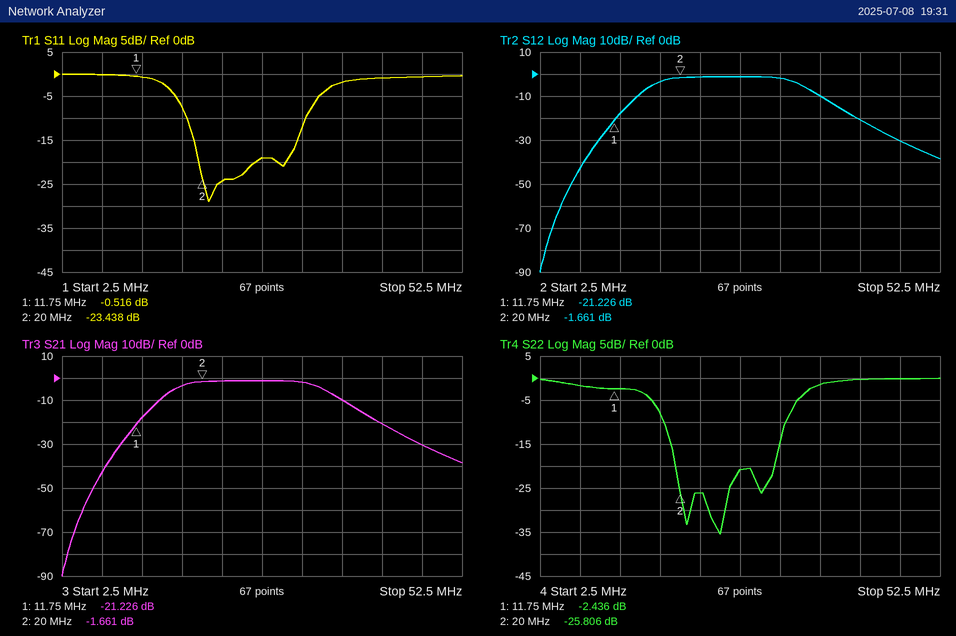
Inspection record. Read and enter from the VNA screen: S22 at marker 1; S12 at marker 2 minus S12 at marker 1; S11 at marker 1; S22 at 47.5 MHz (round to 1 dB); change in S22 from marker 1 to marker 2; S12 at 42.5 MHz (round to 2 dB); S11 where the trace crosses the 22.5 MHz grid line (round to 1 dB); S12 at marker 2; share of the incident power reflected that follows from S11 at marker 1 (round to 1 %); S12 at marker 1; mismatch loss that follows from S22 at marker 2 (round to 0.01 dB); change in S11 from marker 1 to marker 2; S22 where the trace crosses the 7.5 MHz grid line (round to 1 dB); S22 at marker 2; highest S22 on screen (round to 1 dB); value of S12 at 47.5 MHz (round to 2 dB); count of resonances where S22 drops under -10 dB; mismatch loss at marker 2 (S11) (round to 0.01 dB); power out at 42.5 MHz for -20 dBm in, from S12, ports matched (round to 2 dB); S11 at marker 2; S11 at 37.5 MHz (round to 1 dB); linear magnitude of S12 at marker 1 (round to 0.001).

-2.436 dB
19.565 dB
-0.516 dB
0 dB
-23.370 dB
-20 dB
-24 dB
-1.661 dB
89 %
-21.226 dB
0.01 dB
-22.922 dB
-2 dB
-25.806 dB
0 dB
-30 dB
3
0.02 dB
-40 dBm
-23.438 dB
-2 dB
0.087
